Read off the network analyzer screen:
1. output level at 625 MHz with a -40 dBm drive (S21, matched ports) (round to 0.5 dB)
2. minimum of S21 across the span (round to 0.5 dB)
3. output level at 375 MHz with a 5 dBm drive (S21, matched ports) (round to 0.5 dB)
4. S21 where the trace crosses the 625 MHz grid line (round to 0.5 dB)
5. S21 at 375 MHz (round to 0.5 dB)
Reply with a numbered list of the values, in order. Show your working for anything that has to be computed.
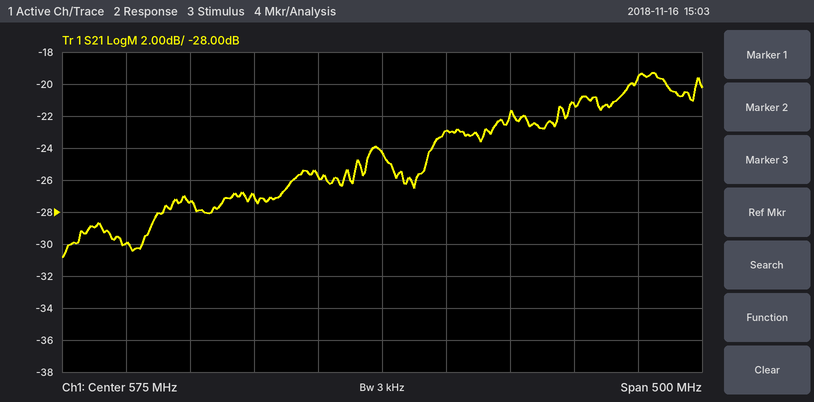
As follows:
1. -40 dBm + (-23.0 dB) = -63.0 dBm
2. -31.0 dB
3. 5 dBm + (-30.0 dB) = -25.0 dBm
4. -23.0 dB
5. -30.0 dB
